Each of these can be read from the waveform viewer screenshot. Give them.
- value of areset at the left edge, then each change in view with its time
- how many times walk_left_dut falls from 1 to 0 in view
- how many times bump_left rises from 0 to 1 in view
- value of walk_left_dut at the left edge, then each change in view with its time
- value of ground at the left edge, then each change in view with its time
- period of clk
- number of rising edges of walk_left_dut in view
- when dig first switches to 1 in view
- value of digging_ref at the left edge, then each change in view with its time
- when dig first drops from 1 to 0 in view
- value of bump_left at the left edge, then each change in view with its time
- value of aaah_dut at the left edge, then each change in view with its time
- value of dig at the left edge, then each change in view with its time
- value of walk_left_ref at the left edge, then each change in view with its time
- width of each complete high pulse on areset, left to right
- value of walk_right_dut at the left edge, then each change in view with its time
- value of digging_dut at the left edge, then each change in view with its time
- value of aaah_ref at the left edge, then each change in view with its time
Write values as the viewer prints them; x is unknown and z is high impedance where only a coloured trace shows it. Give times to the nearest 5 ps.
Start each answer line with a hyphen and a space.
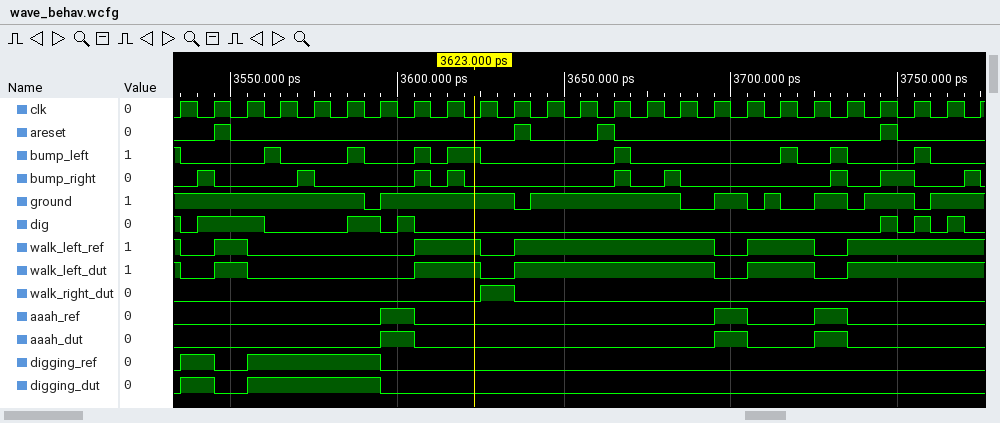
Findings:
- 0, 1 at 3545 ps, 0 at 3550 ps, 1 at 3635 ps, 0 at 3640 ps, 1 at 3660 ps, 0 at 3665 ps, 1 at 3745 ps, 0 at 3750 ps
- 5
- 8
- 1, 0 at 3535 ps, 1 at 3545 ps, 0 at 3555 ps, 1 at 3605 ps, 0 at 3625 ps, 1 at 3635 ps, 0 at 3695 ps, 1 at 3705 ps, 0 at 3725 ps, 1 at 3735 ps
- 1, 0 at 3590 ps, 1 at 3595 ps, 0 at 3635 ps, 1 at 3640 ps, 0 at 3685 ps, 1 at 3695 ps, 0 at 3705 ps, 1 at 3710 ps, 0 at 3715 ps, 1 at 3725 ps, 0 at 3735 ps, 1 at 3740 ps, 0 at 3755 ps, 1 at 3760 ps
- 10 ps
- 5
- 3540 ps
- 0, 1 at 3535 ps, 0 at 3545 ps, 1 at 3555 ps, 0 at 3595 ps
- 3535 ps
- 1, 0 at 3535 ps, 1 at 3560 ps, 0 at 3565 ps, 1 at 3585 ps, 0 at 3590 ps, 1 at 3605 ps, 0 at 3610 ps, 1 at 3615 ps, 0 at 3625 ps, 1 at 3665 ps, 0 at 3670 ps, 1 at 3715 ps, 0 at 3720 ps, 1 at 3730 ps, 0 at 3735 ps, 1 at 3755 ps, 0 at 3760 ps
- 0, 1 at 3595 ps, 0 at 3605 ps, 1 at 3695 ps, 0 at 3705 ps, 1 at 3725 ps, 0 at 3735 ps
- 1, 0 at 3535 ps, 1 at 3540 ps, 0 at 3560 ps, 1 at 3585 ps, 0 at 3595 ps, 1 at 3600 ps, 0 at 3605 ps, 1 at 3745 ps, 0 at 3750 ps, 1 at 3755 ps, 0 at 3760 ps, 1 at 3765 ps, 0 at 3770 ps
- 1, 0 at 3535 ps, 1 at 3545 ps, 0 at 3555 ps, 1 at 3605 ps, 0 at 3625 ps, 1 at 3635 ps, 0 at 3695 ps, 1 at 3705 ps, 0 at 3725 ps, 1 at 3735 ps
- 5 ps, 5 ps, 5 ps, 5 ps
- 0, 1 at 3625 ps, 0 at 3635 ps
- 0, 1 at 3535 ps, 0 at 3545 ps, 1 at 3555 ps, 0 at 3595 ps
- 0, 1 at 3595 ps, 0 at 3605 ps, 1 at 3695 ps, 0 at 3705 ps, 1 at 3725 ps, 0 at 3735 ps
